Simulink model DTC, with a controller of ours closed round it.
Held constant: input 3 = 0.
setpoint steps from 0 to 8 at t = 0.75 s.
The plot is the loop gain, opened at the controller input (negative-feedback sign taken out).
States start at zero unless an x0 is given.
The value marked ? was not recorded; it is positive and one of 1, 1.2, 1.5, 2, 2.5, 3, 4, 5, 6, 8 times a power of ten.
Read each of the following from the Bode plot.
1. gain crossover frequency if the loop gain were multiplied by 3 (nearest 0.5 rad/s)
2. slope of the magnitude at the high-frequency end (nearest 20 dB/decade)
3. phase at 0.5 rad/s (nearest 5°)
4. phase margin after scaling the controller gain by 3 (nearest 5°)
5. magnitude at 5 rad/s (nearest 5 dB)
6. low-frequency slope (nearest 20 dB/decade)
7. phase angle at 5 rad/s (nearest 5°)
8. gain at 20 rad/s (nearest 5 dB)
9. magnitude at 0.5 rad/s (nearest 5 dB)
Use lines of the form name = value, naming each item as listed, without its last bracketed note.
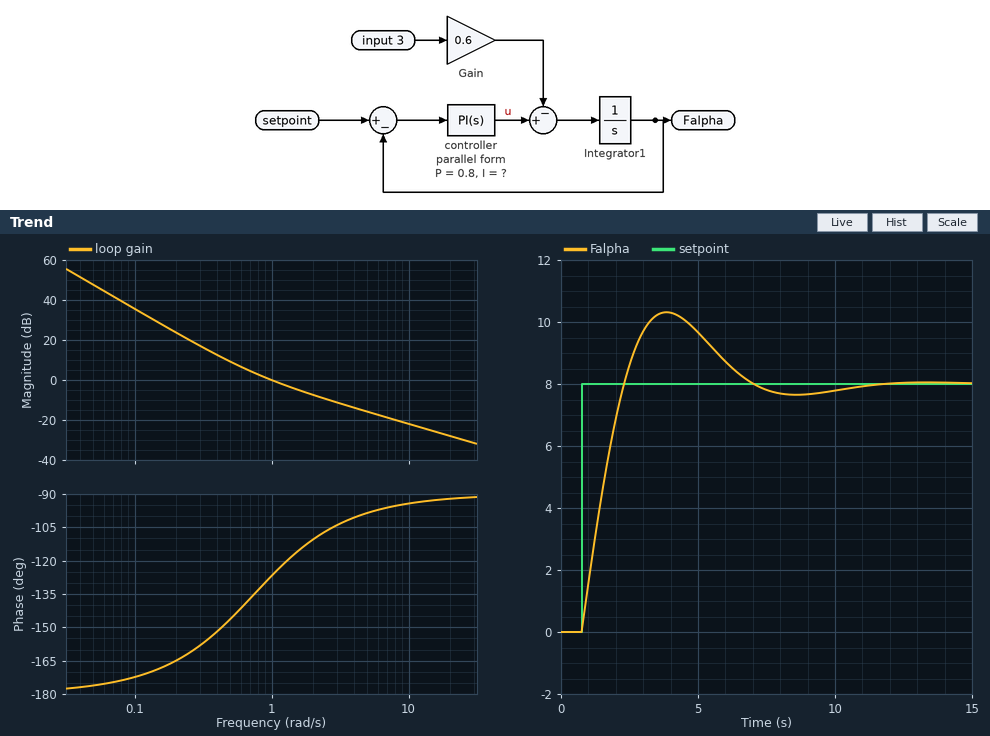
gain crossover frequency if the loop gain were multiplied by 3 = 2.5 rad/s
slope of the magnitude at the high-frequency end = -20 dB/decade
phase at 0.5 rad/s = -145°
phase margin after scaling the controller gain by 3 = 75°
magnitude at 5 rad/s = -15 dB
low-frequency slope = -40 dB/decade
phase angle at 5 rad/s = -100°
gain at 20 rad/s = -30 dB
magnitude at 0.5 rad/s = 10 dB
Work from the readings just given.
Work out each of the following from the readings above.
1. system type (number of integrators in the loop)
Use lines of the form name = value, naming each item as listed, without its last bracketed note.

system type = 2
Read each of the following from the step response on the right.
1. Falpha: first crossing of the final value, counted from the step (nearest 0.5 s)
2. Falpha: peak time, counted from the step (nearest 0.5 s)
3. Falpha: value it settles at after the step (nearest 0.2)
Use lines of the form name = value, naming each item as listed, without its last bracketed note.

Falpha: first crossing of the final value, counted from the step = 1.5 s
Falpha: peak time, counted from the step = 3.0 s
Falpha: value it settles at after the step = 8.0
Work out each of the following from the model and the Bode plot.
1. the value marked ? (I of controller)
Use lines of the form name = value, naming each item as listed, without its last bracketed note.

the value marked ? = 0.6
